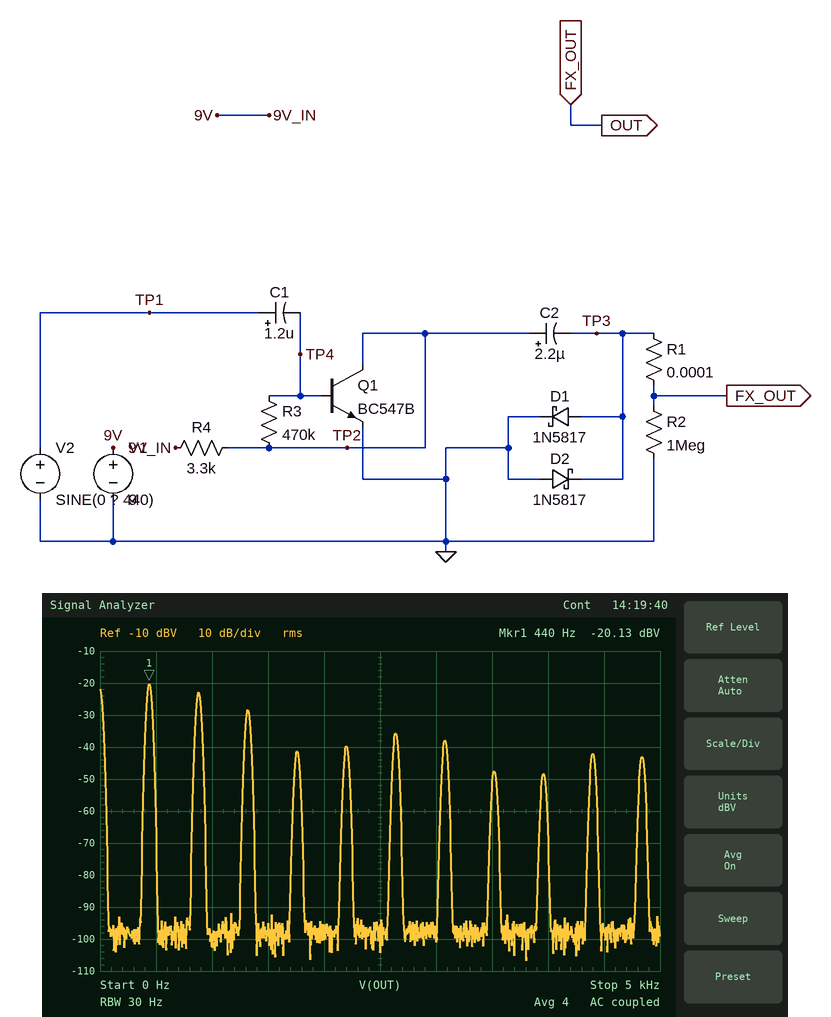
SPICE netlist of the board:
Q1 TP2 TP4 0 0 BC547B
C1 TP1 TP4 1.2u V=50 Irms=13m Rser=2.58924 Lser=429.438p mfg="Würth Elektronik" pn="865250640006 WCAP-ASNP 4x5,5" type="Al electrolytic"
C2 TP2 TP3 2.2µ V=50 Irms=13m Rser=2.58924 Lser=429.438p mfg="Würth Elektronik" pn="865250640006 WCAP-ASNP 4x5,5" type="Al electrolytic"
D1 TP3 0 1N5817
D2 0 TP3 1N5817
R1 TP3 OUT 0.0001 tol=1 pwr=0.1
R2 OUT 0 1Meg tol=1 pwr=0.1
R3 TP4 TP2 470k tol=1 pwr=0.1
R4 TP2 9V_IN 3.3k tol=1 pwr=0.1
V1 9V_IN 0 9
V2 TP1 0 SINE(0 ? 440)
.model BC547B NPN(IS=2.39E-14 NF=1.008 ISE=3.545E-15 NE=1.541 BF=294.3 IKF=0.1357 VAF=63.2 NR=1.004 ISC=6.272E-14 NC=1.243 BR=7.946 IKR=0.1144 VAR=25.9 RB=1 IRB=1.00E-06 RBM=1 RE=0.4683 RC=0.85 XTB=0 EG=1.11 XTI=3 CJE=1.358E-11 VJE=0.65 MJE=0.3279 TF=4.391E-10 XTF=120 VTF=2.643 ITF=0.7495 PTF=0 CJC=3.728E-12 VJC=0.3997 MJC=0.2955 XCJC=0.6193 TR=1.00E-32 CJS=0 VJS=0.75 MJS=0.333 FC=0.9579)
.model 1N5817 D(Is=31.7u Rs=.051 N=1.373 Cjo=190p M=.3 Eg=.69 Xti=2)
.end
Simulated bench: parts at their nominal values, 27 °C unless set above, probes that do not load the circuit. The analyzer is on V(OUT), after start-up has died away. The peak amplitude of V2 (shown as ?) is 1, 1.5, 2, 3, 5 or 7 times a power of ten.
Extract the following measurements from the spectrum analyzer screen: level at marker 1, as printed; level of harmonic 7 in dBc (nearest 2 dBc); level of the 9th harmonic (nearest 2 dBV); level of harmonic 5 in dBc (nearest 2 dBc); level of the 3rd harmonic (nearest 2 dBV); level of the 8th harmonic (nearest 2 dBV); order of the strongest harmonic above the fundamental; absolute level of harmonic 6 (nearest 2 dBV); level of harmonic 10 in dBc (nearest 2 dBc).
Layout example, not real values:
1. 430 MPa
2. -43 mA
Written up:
1. -20.13 dBV
2. -18 dBc
3. -48 dBV
4. -20 dBc
5. -28 dBV
6. -48 dBV
7. 2
8. -36 dBV
9. -22 dBc
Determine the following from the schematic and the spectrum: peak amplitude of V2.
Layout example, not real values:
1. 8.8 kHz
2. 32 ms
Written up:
1. 200 mV
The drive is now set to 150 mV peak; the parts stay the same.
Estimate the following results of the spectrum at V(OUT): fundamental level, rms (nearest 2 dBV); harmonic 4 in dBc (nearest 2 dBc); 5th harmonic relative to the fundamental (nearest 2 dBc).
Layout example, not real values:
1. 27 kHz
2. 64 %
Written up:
1. -20 dBV
2. -36 dBc
3. -16 dBc
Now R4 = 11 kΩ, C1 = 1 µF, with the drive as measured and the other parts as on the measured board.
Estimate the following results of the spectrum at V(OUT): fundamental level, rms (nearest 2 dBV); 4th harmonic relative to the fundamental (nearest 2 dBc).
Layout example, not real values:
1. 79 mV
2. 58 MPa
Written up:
1. -22 dBV
2. -18 dBc
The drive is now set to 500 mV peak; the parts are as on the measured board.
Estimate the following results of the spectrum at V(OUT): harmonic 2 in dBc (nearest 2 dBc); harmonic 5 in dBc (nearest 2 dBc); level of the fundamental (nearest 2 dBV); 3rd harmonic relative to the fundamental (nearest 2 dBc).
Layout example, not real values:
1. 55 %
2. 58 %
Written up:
1. -2 dBc
2. -14 dBc
3. -22 dBV
4. -4 dBc
